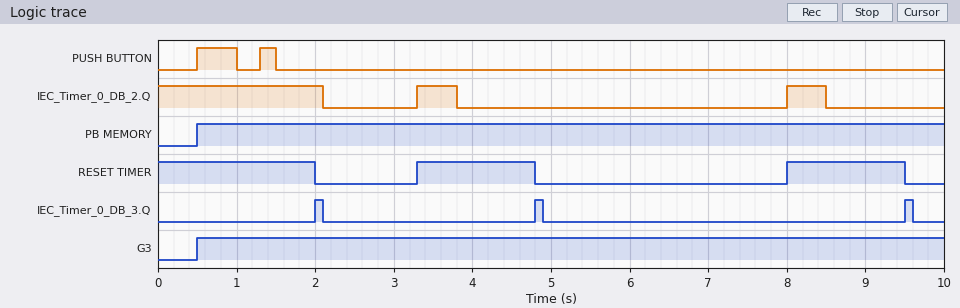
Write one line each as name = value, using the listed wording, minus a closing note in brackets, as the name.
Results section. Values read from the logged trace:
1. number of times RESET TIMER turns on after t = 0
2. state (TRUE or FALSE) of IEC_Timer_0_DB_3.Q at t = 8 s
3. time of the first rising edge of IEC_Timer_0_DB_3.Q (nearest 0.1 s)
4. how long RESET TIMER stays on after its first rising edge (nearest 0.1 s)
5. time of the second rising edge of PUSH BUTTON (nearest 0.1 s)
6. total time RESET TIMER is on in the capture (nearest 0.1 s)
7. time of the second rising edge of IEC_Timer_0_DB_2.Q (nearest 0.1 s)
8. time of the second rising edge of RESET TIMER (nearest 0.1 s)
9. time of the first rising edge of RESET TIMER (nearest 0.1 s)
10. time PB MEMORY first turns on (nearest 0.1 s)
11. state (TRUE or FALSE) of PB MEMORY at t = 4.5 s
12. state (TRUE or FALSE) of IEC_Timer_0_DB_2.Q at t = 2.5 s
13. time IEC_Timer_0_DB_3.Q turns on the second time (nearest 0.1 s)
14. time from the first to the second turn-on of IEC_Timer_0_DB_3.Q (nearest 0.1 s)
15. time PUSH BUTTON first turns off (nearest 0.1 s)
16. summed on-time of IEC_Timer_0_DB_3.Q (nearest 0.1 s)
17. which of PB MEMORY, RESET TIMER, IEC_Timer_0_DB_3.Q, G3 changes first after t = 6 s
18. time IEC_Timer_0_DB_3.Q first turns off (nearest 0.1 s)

number of times RESET TIMER turns on after t = 0 = 2
state (TRUE or FALSE) of IEC_Timer_0_DB_3.Q at t = 8 s = FALSE
time of the first rising edge of IEC_Timer_0_DB_3.Q = 2.0 s
how long RESET TIMER stays on after its first rising edge = 1.5 s
time of the second rising edge of PUSH BUTTON = 1.3 s
total time RESET TIMER is on in the capture = 5.0 s
time of the second rising edge of IEC_Timer_0_DB_2.Q = 8.0 s
time of the second rising edge of RESET TIMER = 8.0 s
time of the first rising edge of RESET TIMER = 3.3 s
time PB MEMORY first turns on = 0.5 s
state (TRUE or FALSE) of PB MEMORY at t = 4.5 s = TRUE
state (TRUE or FALSE) of IEC_Timer_0_DB_2.Q at t = 2.5 s = FALSE
time IEC_Timer_0_DB_3.Q turns on the second time = 4.8 s
time from the first to the second turn-on of IEC_Timer_0_DB_3.Q = 2.8 s
time PUSH BUTTON first turns off = 1.0 s
summed on-time of IEC_Timer_0_DB_3.Q = 0.3 s
which of PB MEMORY, RESET TIMER, IEC_Timer_0_DB_3.Q, G3 changes first after t = 6 s = RESET TIMER
time IEC_Timer_0_DB_3.Q first turns off = 2.1 s
